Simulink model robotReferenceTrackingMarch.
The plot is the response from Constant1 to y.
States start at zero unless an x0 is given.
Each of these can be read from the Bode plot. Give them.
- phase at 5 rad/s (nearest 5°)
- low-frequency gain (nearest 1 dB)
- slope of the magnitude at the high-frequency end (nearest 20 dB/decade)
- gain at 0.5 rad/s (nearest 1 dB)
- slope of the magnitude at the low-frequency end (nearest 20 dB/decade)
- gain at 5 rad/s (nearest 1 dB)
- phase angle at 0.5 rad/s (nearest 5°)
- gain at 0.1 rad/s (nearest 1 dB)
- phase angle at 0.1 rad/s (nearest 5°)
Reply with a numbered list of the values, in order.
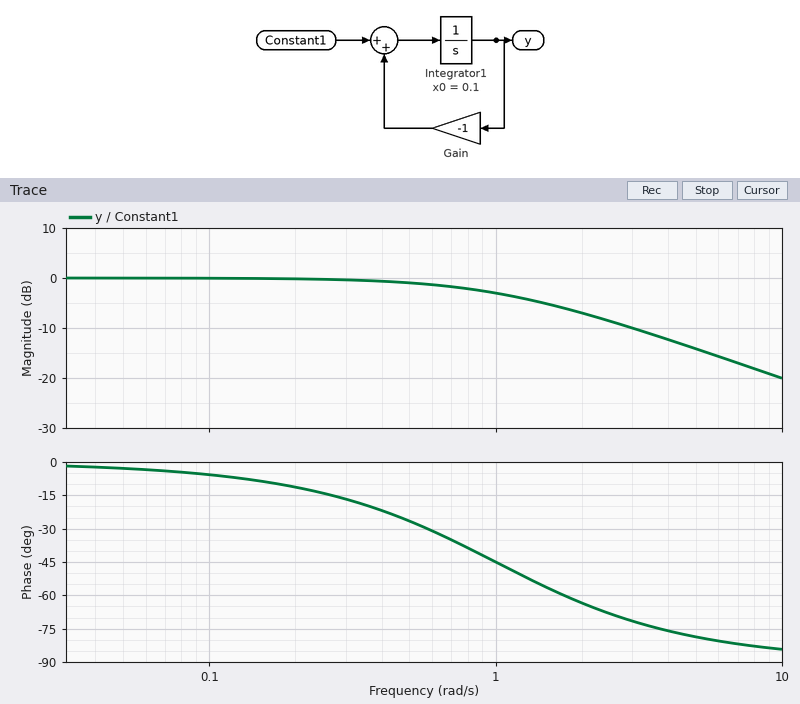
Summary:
1. -80°
2. 0 dB
3. -20 dB/decade
4. -1 dB
5. 0 dB/decade
6. -14 dB
7. -25°
8. 0 dB
9. -5°
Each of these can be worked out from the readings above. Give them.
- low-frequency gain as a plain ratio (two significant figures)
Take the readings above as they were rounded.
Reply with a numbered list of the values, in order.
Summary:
1. 1.0
